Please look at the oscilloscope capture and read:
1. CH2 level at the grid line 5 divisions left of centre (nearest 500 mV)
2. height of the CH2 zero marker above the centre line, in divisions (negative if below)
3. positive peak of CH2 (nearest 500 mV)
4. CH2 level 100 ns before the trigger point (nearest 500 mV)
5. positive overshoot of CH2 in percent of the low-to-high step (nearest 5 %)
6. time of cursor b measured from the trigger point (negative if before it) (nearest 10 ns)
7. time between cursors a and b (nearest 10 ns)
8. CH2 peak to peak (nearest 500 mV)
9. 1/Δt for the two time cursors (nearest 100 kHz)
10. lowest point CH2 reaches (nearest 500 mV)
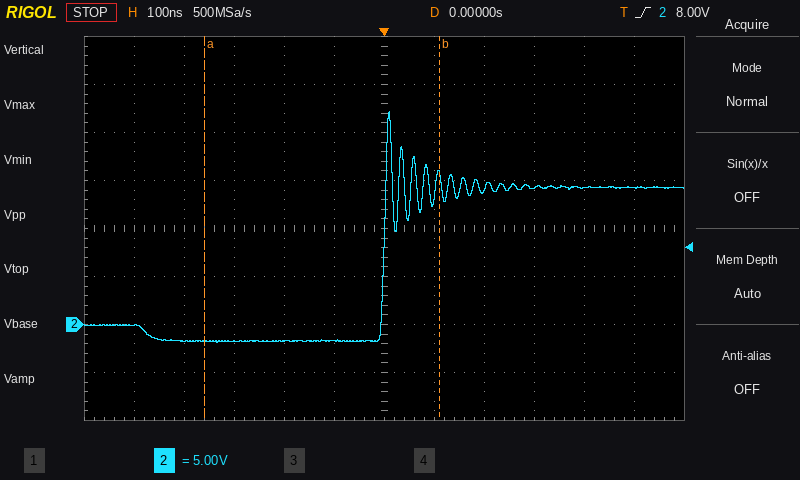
0.0 V
-2.0 div
22.0 V
-1.5 V
50 %
+110 ns
470 ns
24.0 V
2.1 MHz
-2.0 V
